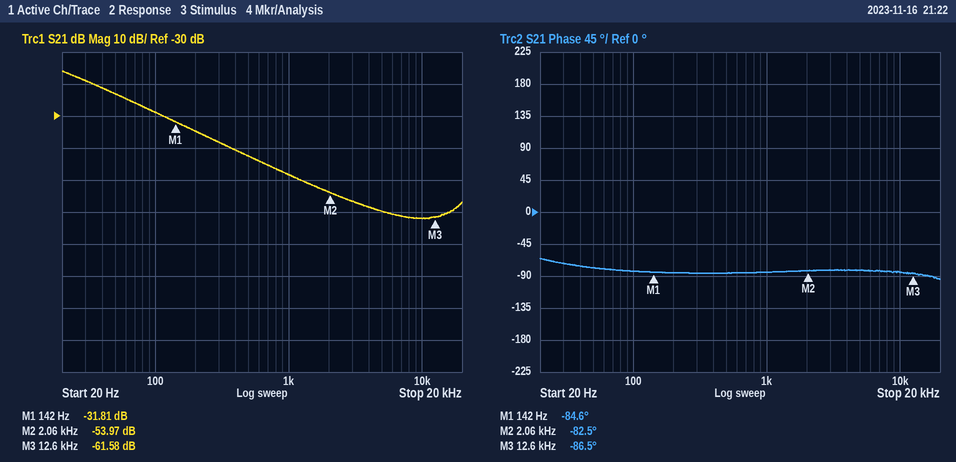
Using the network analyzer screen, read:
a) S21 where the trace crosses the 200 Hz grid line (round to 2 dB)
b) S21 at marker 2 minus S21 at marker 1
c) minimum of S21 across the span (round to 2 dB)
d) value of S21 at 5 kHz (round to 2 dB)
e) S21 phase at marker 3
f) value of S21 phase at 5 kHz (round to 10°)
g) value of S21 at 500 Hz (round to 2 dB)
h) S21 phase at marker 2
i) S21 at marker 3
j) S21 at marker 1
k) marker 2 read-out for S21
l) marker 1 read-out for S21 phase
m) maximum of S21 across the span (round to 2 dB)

-34 dB
-22.16 dB
-62 dB
-60 dB
-86.5°
-80°
-42 dB
-82.5°
-61.58 dB
-31.81 dB
-53.97 dB
-84.6°
-16 dB
